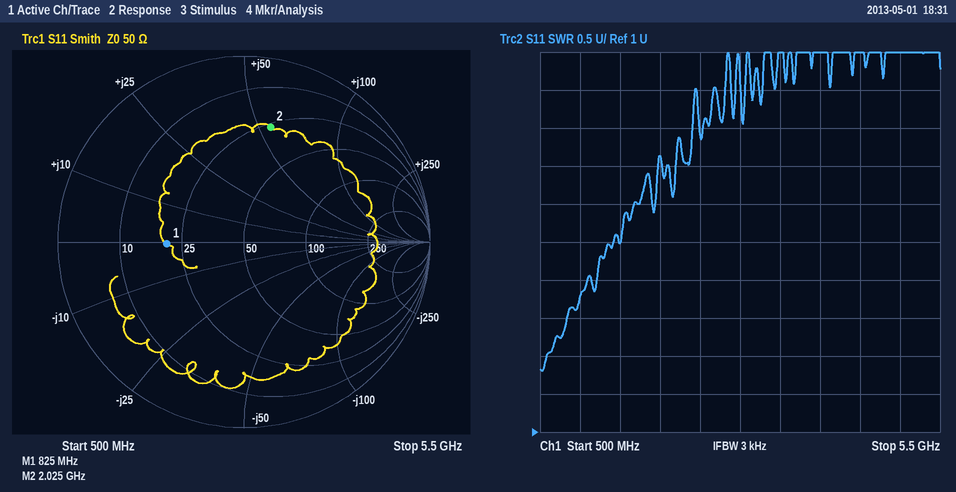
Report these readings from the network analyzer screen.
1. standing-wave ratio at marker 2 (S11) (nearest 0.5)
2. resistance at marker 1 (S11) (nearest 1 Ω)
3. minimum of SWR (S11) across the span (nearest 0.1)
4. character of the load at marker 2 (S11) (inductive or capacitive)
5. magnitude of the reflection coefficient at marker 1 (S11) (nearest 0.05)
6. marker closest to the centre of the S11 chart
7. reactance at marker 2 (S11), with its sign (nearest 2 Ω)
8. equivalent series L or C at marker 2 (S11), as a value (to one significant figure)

4.5
21 Ω
1.8
inductive
0.40
marker 1
+56 Ω
4 nH
